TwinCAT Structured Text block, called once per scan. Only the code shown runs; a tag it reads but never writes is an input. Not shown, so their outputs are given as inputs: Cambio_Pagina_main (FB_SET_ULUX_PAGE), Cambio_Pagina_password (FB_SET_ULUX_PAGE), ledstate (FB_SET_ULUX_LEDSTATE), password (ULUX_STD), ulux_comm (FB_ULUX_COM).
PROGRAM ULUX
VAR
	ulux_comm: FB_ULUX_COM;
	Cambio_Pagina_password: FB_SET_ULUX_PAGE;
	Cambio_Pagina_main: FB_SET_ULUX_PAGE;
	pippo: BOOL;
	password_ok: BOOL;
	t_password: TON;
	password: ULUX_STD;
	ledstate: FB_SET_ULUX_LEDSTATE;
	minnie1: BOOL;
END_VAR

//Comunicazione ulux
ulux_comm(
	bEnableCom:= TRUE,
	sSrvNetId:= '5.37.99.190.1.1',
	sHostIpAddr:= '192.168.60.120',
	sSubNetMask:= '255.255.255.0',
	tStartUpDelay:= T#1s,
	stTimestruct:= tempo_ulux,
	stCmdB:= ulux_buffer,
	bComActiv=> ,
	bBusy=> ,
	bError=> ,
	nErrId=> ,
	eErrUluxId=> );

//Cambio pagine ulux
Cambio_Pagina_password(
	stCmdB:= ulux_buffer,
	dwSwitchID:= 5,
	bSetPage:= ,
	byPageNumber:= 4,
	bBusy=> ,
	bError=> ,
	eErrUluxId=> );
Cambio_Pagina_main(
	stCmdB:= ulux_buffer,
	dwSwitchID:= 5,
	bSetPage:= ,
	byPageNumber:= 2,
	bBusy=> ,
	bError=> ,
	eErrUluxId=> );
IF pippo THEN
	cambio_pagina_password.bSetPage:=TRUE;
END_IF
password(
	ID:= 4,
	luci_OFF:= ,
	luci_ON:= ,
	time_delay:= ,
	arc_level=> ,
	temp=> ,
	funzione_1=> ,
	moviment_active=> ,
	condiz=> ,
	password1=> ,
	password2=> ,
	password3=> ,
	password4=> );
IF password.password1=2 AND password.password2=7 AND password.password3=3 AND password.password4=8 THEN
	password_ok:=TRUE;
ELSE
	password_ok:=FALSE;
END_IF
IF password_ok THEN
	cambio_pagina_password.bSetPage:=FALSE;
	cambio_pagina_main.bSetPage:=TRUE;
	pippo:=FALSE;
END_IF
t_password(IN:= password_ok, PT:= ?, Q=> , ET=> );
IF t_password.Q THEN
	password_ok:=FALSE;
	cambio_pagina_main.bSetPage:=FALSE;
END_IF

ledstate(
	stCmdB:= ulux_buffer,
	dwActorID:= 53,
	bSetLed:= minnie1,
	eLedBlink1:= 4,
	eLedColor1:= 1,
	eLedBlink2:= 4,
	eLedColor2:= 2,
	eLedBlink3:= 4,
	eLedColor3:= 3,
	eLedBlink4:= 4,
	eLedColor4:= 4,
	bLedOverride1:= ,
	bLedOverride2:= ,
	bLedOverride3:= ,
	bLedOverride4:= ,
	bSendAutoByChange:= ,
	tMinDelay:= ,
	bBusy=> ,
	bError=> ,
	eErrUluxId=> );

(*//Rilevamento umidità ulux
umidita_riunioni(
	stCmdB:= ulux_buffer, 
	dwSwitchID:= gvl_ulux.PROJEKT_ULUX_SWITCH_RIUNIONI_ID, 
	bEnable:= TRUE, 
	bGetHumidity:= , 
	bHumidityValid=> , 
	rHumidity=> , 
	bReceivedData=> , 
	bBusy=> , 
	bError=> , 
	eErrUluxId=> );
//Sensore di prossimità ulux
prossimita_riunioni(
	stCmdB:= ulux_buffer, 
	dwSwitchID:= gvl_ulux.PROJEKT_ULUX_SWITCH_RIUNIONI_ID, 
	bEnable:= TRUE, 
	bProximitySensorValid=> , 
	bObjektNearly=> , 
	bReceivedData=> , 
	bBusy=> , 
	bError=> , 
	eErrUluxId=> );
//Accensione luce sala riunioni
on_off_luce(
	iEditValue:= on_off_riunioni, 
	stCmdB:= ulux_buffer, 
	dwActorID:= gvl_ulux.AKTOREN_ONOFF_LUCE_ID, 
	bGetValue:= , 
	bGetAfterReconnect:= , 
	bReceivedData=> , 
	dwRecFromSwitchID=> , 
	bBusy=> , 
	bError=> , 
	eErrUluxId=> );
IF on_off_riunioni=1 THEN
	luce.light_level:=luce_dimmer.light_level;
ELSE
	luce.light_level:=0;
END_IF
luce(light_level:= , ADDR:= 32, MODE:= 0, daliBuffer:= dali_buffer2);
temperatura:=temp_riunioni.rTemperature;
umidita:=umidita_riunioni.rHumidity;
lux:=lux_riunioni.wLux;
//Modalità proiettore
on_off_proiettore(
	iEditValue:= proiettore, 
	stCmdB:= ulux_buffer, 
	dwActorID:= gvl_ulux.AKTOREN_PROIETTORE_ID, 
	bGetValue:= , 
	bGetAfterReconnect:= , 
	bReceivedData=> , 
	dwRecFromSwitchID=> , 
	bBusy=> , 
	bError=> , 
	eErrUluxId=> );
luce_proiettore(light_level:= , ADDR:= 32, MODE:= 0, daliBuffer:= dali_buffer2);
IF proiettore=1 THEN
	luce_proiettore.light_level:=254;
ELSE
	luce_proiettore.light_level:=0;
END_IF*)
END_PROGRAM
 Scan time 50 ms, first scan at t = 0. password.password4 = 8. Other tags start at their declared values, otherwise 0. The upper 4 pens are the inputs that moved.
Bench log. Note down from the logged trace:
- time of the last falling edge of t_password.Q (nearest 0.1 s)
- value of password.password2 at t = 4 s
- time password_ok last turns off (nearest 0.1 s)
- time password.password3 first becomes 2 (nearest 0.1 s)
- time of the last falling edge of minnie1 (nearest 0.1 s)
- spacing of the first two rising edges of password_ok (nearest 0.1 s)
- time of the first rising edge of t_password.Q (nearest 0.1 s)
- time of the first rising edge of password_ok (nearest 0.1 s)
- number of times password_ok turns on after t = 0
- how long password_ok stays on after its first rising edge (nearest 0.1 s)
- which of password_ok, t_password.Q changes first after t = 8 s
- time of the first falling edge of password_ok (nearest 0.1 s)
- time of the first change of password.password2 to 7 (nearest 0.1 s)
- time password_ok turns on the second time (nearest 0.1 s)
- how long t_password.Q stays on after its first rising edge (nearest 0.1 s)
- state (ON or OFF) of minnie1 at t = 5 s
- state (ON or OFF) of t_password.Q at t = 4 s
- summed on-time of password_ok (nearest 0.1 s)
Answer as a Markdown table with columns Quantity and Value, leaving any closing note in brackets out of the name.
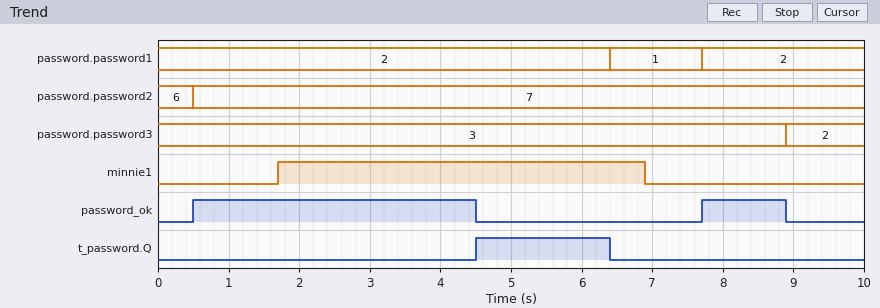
| Quantity | Value |
|---|---|
| time of the last falling edge of t_password.Q | 6.4 s |
| value of password.password2 at t = 4 s | 7 |
| time password_ok last turns off | 8.9 s |
| time password.password3 first becomes 2 | 8.9 s |
| time of the last falling edge of minnie1 | 6.9 s |
| spacing of the first two rising edges of password_ok | 7.2 s |
| time of the first rising edge of t_password.Q | 4.5 s |
| time of the first rising edge of password_ok | 0.5 s |
| number of times password_ok turns on after t = 0 | 2 |
| how long password_ok stays on after its first rising edge | 4.0 s |
| which of password_ok, t_password.Q changes first after t = 8 s | password_ok |
| time of the first falling edge of password_ok | 4.5 s |
| time of the first change of password.password2 to 7 | 0.5 s |
| time password_ok turns on the second time | 7.7 s |
| how long t_password.Q stays on after its first rising edge | 1.9 s |
| state (ON or OFF) of minnie1 at t = 5 s | ON |
| state (ON or OFF) of t_password.Q at t = 4 s | OFF |
| summed on-time of password_ok | 5.2 s |
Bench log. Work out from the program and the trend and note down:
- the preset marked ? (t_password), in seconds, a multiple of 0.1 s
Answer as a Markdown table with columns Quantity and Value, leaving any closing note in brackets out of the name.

| Quantity | Value |
|---|---|
| the preset marked ? (t_password), in seconds, a multiple of 0.1 s | 4.0 s |
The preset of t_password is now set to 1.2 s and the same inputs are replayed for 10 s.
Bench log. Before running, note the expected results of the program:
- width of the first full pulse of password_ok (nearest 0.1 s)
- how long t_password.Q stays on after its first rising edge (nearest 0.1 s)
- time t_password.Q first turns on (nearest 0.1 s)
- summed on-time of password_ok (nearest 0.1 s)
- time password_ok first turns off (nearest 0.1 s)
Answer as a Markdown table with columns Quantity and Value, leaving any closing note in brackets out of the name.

| Quantity | Value |
|---|---|
| width of the first full pulse of password_ok | 1.2 s |
| how long t_password.Q stays on after its first rising edge | 4.7 s |
| time t_password.Q first turns on | 1.7 s |
| summed on-time of password_ok | 2.4 s |
| time password_ok first turns off | 1.7 s |
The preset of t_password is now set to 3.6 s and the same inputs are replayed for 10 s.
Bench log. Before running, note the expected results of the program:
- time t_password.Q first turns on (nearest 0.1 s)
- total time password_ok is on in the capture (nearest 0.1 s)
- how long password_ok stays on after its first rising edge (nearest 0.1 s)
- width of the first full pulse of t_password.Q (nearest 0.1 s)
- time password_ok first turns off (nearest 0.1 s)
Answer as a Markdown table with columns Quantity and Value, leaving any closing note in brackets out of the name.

| Quantity | Value |
|---|---|
| time t_password.Q first turns on | 4.1 s |
| total time password_ok is on in the capture | 4.8 s |
| how long password_ok stays on after its first rising edge | 3.6 s |
| width of the first full pulse of t_password.Q | 2.3 s |
| time password_ok first turns off | 4.1 s |
